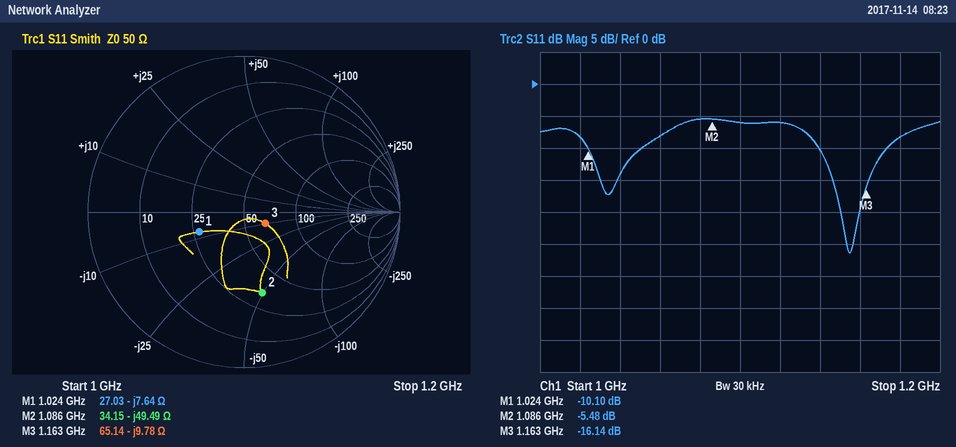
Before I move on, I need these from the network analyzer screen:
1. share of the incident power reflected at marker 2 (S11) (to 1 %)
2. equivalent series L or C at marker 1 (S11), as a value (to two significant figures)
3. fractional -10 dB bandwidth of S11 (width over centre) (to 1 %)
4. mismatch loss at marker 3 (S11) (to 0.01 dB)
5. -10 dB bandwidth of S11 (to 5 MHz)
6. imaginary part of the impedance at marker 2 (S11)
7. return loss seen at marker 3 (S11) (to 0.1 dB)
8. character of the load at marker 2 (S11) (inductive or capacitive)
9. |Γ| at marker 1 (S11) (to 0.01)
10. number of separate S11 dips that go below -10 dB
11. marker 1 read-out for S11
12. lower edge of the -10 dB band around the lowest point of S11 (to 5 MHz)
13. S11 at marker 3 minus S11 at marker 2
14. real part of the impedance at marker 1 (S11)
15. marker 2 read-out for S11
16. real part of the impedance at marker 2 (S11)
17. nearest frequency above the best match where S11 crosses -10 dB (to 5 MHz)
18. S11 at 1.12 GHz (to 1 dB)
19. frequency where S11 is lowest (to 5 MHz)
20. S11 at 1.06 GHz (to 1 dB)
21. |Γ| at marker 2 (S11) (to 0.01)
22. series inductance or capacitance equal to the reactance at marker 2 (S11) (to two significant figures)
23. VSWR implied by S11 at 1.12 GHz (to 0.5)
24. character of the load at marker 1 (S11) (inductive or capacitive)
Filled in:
28 %
20 pF
3 %
0.11 dB
35 MHz
-49.49 Ω
16.1 dB
capacitive
0.31
2
-10.10 dB
1.140 GHz
-10.66 dB
27.03 Ω
-5.48 dB
34.15 Ω
1.175 GHz
-6 dB
1.155 GHz
-8 dB
0.53
3.0 pF
3.0
capacitive
